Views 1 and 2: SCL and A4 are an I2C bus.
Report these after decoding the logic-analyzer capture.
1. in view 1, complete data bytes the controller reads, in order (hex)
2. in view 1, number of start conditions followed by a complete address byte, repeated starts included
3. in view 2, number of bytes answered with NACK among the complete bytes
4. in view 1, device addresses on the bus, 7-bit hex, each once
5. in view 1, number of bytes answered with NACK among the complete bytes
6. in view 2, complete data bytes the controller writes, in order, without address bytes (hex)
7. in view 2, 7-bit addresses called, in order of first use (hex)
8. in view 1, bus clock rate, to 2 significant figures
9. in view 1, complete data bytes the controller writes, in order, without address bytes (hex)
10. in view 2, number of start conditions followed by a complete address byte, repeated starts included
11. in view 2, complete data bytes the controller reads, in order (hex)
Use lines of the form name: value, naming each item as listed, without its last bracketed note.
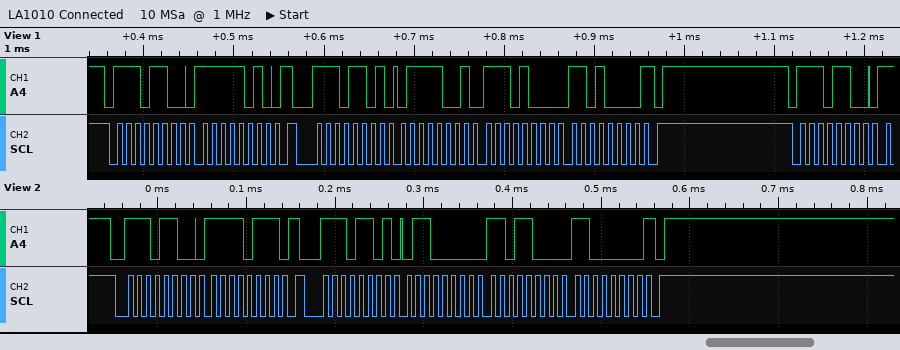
in view 1, complete data bytes the controller reads, in order: 79 E8 D0
in view 1, number of start conditions followed by a complete address byte, repeated starts included: 3
in view 2, number of bytes answered with NACK among the complete bytes: 1
in view 1, device addresses on the bus, 7-bit hex, each once: 0x76
in view 1, number of bytes answered with NACK among the complete bytes: 1
in view 2, complete data bytes the controller writes, in order, without address bytes: F7
in view 2, 7-bit addresses called, in order of first use: 0x76
in view 1, bus clock rate, to 2 significant figures: 100 kHz
in view 1, complete data bytes the controller writes, in order, without address bytes: FA
in view 2, number of start conditions followed by a complete address byte, repeated starts included: 2
in view 2, complete data bytes the controller reads, in order: 60 D8 C0
